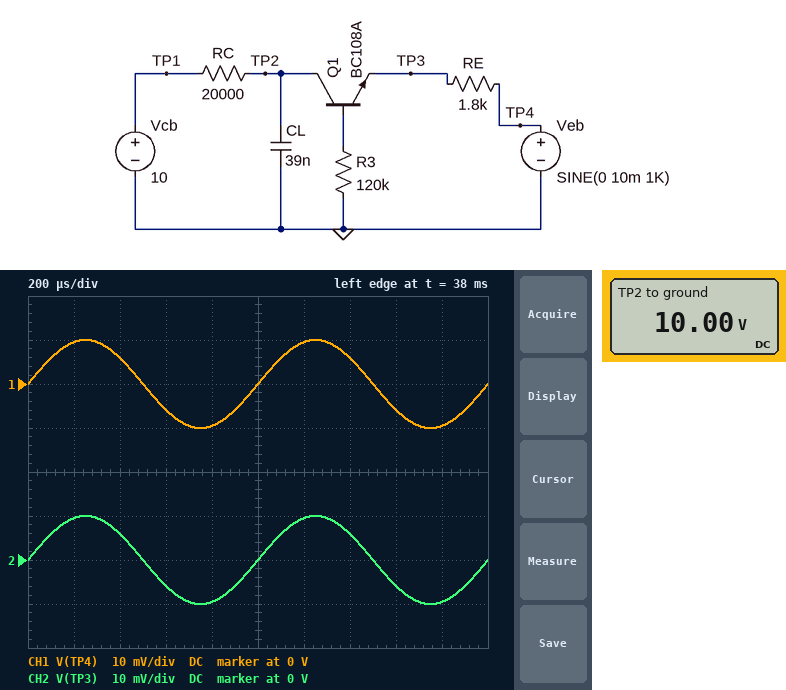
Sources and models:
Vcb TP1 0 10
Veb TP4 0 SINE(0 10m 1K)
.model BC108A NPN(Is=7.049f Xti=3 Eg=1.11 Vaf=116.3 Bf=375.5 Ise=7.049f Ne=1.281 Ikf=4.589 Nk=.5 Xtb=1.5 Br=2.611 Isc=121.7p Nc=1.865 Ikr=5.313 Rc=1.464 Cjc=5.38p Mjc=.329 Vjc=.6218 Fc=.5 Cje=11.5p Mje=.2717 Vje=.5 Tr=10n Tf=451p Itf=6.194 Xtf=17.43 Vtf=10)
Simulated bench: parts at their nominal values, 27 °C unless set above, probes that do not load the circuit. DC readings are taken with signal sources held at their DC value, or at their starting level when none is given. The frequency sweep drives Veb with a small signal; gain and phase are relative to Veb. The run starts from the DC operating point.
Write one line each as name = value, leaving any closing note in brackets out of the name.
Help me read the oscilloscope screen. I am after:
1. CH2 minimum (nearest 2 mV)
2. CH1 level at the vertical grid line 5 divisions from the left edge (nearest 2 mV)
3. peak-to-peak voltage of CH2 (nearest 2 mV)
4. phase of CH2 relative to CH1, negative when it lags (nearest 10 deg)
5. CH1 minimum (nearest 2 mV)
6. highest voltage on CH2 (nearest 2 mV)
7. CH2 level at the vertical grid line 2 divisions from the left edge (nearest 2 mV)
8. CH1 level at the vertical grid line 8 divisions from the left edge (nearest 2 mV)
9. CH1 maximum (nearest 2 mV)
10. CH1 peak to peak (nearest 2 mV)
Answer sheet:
CH2 minimum = -10 mV
CH1 level at the vertical grid line 5 divisions from the left edge = 0 V
peak-to-peak voltage of CH2 = 20 mV
phase of CH2 relative to CH1, negative when it lags = 0 deg
CH1 minimum = -10 mV
highest voltage on CH2 = 10 mV
CH2 level at the vertical grid line 2 divisions from the left edge = 6 mV
CH1 level at the vertical grid line 8 divisions from the left edge = -6 mV
CH1 maximum = 10 mV
CH1 peak to peak = 20 mV
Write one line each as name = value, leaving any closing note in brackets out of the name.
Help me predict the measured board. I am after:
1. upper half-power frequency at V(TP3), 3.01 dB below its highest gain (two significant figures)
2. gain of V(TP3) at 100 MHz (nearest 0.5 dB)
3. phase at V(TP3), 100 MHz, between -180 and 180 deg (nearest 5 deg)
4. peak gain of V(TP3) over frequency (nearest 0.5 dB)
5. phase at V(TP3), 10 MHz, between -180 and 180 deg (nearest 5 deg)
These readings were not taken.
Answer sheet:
upper half-power frequency at V(TP3), 3.01 dB below its highest gain = 49 MHz
gain of V(TP3) at 100 MHz = -7.0 dB
phase at V(TP3), 100 MHz, between -180 and 180 deg = -65 deg
peak gain of V(TP3) over frequency = 0 dB
phase at V(TP3), 10 MHz, between -180 and 180 deg = -10 deg
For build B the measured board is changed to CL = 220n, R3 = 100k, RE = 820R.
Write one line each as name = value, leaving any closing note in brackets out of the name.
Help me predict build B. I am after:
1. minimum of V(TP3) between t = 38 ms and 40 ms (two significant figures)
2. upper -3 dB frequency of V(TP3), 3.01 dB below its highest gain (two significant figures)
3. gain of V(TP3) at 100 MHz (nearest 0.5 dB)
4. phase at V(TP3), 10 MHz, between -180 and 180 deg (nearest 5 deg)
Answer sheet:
minimum of V(TP3) between t = 38 ms and 40 ms = -10 mV
upper -3 dB frequency of V(TP3), 3.01 dB below its highest gain = 110 MHz
gain of V(TP3) at 100 MHz = -2.5 dB
phase at V(TP3), 10 MHz, between -180 and 180 deg = -5 deg
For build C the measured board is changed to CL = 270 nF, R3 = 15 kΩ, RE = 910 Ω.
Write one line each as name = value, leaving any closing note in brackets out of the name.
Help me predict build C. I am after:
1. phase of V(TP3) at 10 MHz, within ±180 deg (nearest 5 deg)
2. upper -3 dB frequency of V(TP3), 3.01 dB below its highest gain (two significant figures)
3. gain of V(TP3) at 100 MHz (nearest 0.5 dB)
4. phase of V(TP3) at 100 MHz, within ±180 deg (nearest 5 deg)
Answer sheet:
phase of V(TP3) at 10 MHz, within ±180 deg = -5 deg
upper -3 dB frequency of V(TP3), 3.01 dB below its highest gain = 93 MHz
gain of V(TP3) at 100 MHz = -3.5 dB
phase of V(TP3) at 100 MHz, within ±180 deg = -45 deg
